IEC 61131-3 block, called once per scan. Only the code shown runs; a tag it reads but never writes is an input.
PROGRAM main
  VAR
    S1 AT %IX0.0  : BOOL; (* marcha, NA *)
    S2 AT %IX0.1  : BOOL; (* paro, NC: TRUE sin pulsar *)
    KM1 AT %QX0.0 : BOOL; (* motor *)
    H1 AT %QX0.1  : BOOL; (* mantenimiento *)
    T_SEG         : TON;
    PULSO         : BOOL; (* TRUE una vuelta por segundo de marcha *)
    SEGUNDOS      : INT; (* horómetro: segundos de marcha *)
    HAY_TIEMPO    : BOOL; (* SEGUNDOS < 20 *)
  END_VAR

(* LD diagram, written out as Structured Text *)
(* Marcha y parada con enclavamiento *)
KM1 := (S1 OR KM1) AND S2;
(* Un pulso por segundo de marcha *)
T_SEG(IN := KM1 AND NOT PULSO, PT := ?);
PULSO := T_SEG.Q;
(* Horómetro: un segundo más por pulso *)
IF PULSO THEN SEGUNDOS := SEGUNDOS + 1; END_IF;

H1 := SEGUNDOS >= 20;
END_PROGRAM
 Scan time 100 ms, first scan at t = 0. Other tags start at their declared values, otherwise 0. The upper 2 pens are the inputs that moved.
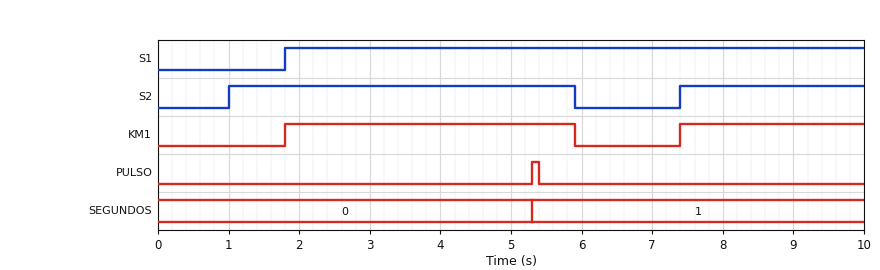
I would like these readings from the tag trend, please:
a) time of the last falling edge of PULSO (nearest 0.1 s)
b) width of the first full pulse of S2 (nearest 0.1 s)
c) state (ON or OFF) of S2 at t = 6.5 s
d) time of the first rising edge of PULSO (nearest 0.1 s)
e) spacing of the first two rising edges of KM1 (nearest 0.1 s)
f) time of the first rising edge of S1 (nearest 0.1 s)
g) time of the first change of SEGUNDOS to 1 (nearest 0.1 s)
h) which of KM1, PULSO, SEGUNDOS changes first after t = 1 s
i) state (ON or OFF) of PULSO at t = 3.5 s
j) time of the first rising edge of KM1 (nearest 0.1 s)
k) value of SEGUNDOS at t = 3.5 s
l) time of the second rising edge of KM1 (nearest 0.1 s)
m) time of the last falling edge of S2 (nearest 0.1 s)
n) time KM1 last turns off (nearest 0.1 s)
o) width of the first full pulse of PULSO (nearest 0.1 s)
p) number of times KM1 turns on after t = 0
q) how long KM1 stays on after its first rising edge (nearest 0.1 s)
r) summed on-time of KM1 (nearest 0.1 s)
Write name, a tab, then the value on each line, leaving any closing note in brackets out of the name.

time of the last falling edge of PULSO	5.4 s
width of the first full pulse of S2	4.9 s
state (ON or OFF) of S2 at t = 6.5 s	OFF
time of the first rising edge of PULSO	5.3 s
spacing of the first two rising edges of KM1	5.6 s
time of the first rising edge of S1	1.8 s
time of the first change of SEGUNDOS to 1	5.3 s
which of KM1, PULSO, SEGUNDOS changes first after t = 1 s	KM1
state (ON or OFF) of PULSO at t = 3.5 s	OFF
time of the first rising edge of KM1	1.8 s
value of SEGUNDOS at t = 3.5 s	0
time of the second rising edge of KM1	7.4 s
time of the last falling edge of S2	5.9 s
time KM1 last turns off	5.9 s
width of the first full pulse of PULSO	0.1 s
number of times KM1 turns on after t = 0	2
how long KM1 stays on after its first rising edge	4.1 s
summed on-time of KM1	6.7 s
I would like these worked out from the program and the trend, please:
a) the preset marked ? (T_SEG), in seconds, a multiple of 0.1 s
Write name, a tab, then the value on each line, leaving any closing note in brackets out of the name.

the preset marked ? (T_SEG), in seconds, a multiple of 0.1 s	3.5 s
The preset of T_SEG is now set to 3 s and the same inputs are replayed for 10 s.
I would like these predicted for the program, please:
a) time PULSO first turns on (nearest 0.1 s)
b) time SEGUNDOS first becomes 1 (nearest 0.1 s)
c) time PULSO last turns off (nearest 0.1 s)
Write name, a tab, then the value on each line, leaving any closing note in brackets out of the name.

time PULSO first turns on	4.8 s
time SEGUNDOS first becomes 1	4.8 s
time PULSO last turns off	4.9 s
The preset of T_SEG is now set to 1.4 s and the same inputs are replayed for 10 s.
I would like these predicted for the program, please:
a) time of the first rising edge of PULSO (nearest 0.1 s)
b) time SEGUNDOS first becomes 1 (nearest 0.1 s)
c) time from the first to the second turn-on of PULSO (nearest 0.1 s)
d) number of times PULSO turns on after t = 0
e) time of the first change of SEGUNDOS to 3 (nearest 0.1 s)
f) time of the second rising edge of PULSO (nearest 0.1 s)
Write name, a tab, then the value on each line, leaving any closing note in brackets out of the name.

time of the first rising edge of PULSO	3.2 s
time SEGUNDOS first becomes 1	3.2 s
time from the first to the second turn-on of PULSO	1.6 s
number of times PULSO turns on after t = 0	3
time of the first change of SEGUNDOS to 3	8.8 s
time of the second rising edge of PULSO	4.8 s
